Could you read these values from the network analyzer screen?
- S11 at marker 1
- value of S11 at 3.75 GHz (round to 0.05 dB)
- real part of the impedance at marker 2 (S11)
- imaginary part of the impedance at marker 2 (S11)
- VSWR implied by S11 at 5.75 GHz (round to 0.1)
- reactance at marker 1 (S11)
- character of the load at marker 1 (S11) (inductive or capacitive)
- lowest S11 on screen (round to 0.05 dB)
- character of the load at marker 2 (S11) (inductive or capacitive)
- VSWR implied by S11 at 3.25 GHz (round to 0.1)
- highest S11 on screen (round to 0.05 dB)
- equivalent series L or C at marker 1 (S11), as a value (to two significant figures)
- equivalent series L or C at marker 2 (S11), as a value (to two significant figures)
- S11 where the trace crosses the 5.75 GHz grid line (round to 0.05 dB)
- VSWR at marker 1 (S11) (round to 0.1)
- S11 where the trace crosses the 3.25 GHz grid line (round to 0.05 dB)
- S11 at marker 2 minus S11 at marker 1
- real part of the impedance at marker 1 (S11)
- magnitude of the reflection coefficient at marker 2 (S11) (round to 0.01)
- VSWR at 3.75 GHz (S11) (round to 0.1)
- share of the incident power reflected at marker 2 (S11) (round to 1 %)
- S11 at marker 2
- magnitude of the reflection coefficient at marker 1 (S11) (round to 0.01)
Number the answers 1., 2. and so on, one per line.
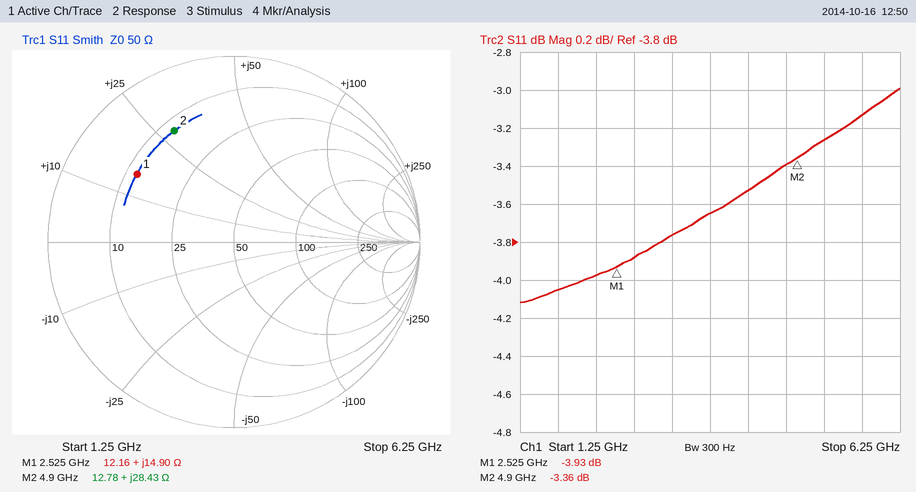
1. -3.93 dB
2. -3.65 dB
3. 12.78 Ω
4. +28.43 Ω
5. 5.6
6. +14.90 Ω
7. inductive
8. -4.10 dB
9. inductive
10. 4.7
11. -3.00 dB
12. 940 pH
13. 920 pH
14. -3.15 dB
15. 4.5
16. -3.75 dB
17. 0.57 dB
18. 12.16 Ω
19. 0.68
20. 4.8
21. 46 %
22. -3.36 dB
23. 0.64
